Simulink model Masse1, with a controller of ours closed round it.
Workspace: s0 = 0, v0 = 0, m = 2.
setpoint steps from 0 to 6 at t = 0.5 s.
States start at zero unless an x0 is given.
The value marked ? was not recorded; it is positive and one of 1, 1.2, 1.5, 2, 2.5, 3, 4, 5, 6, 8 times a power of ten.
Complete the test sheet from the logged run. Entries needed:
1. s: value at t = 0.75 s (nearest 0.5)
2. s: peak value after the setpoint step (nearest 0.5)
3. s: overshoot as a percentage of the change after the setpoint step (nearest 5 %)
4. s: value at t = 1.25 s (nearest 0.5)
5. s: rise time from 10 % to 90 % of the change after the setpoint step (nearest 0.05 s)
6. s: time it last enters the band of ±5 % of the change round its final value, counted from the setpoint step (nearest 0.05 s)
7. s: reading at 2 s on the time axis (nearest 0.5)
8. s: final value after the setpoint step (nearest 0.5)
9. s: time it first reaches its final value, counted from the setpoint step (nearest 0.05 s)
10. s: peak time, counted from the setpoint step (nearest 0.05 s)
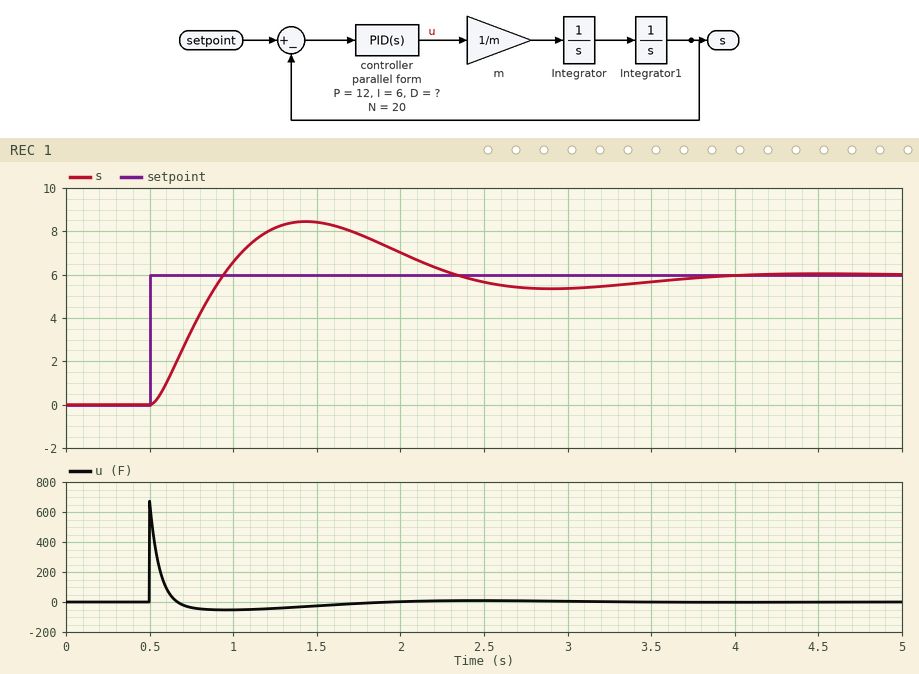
3.5
8.5
40 %
8.0
0.30 s
3.05 s
7.0
6.0
0.45 s
0.95 s
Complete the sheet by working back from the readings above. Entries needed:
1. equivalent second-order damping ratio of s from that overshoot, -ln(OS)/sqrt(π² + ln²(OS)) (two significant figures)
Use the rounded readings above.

0.28
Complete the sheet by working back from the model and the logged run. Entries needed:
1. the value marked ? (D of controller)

5
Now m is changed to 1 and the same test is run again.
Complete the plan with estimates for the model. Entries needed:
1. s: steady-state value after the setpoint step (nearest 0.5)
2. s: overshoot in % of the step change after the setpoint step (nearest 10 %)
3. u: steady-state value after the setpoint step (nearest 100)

6.0
30 %
0
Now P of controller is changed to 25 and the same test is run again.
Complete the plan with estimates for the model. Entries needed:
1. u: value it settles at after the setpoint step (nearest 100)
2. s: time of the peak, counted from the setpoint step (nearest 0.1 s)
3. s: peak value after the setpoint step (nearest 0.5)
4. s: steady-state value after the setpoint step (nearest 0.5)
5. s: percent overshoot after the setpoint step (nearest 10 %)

0
0.7 s
9.0
6.0
50 %
